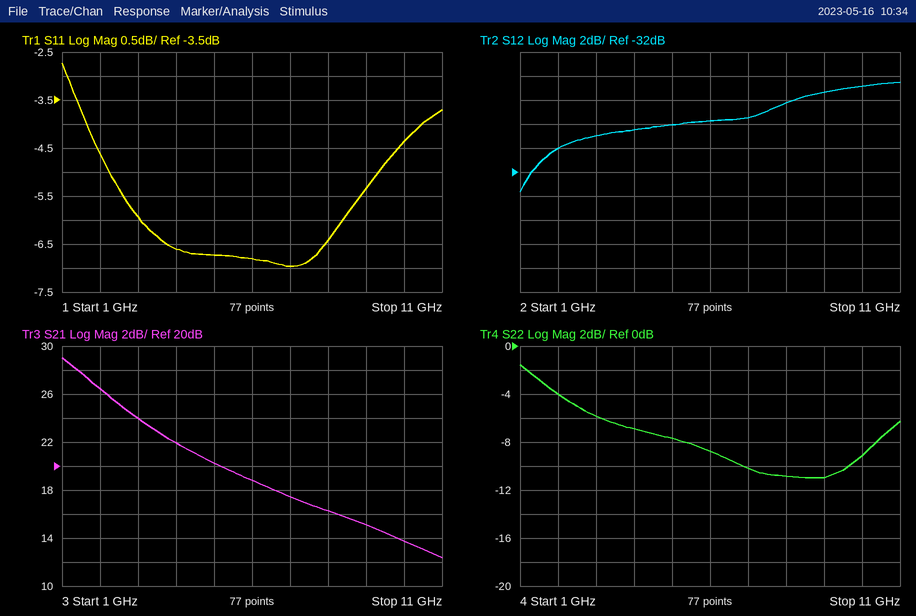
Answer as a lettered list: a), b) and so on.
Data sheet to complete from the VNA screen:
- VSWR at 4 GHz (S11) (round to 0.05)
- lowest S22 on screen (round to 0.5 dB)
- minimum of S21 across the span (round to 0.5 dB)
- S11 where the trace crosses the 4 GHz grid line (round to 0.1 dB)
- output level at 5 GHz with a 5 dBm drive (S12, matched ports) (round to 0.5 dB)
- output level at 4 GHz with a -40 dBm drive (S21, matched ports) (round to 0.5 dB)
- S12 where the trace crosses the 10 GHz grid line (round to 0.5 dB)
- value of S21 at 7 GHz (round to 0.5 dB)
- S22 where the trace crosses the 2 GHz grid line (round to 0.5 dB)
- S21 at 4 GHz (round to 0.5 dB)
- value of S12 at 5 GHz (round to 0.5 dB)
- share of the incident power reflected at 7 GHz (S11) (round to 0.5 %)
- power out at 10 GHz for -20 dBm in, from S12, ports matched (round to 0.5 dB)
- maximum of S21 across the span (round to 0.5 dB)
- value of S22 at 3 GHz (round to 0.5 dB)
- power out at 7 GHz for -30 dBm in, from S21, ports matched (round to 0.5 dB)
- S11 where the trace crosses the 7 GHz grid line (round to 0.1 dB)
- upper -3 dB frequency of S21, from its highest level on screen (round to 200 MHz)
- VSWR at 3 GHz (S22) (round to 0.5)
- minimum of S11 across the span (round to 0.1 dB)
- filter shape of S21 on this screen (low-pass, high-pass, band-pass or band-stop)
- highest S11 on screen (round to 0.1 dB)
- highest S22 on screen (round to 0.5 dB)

a) 2.75
b) -11.0 dB
c) 12.5 dB
d) -6.6 dB
e) -23.0 dBm
f) -18.0 dBm
g) -25.0 dB
h) 17.5 dB
i) -4.0 dB
j) 22.0 dB
k) -28.0 dB
l) 20.0 %
m) -45.0 dBm
n) 29.0 dB
o) -6.0 dB
p) -12.5 dBm
q) -7.0 dB
r) 2.2 GHz
s) 3.0
t) -7.0 dB
u) low-pass
v) -2.7 dB
w) -1.5 dB
